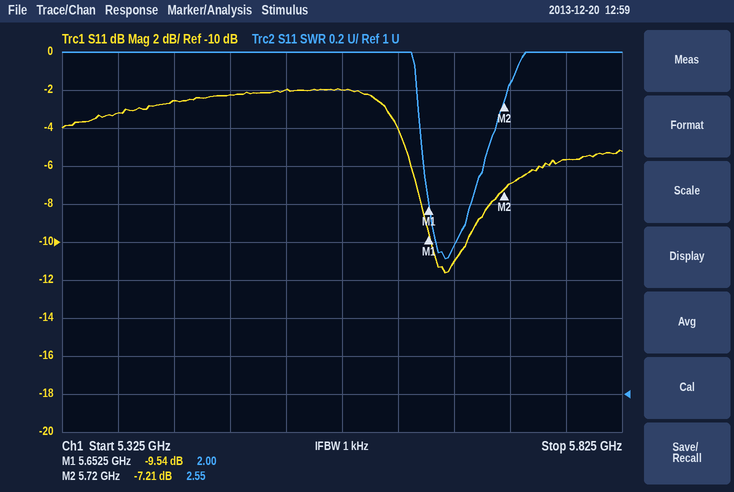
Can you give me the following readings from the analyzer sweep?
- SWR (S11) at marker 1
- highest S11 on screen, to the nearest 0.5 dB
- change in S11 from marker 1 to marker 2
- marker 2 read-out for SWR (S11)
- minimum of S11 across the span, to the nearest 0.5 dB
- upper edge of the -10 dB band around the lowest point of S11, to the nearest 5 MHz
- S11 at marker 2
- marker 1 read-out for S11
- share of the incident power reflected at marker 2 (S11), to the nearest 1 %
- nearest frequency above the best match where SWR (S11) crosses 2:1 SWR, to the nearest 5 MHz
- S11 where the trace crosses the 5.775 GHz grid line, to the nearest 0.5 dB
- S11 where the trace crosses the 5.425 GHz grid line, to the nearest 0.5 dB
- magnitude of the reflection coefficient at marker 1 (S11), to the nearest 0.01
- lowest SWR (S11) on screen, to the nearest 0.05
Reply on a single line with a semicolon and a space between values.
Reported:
2.00; -2.0 dB; 2.33 dB; 2.55; -11.5 dB; 5.685 GHz; -7.21 dB; -9.54 dB; 19 %; 5.690 GHz; -5.5 dB; -2.5 dB; 0.33; 1.70
